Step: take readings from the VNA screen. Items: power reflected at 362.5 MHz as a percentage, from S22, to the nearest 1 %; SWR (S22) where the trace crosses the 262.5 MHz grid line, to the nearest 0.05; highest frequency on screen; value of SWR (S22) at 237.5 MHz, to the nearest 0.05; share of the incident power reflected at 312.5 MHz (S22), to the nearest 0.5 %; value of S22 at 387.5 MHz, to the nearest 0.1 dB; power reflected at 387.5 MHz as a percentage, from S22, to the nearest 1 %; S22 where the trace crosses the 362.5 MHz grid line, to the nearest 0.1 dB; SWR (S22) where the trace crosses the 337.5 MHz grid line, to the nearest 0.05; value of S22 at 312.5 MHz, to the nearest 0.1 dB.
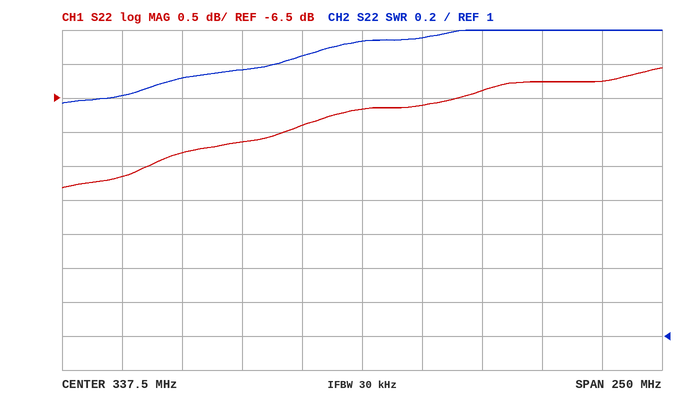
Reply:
22 %
2.50
462.5 MHz
2.40
20.5 %
-6.4 dB
23 %
-6.6 dB
2.75
-6.9 dB
